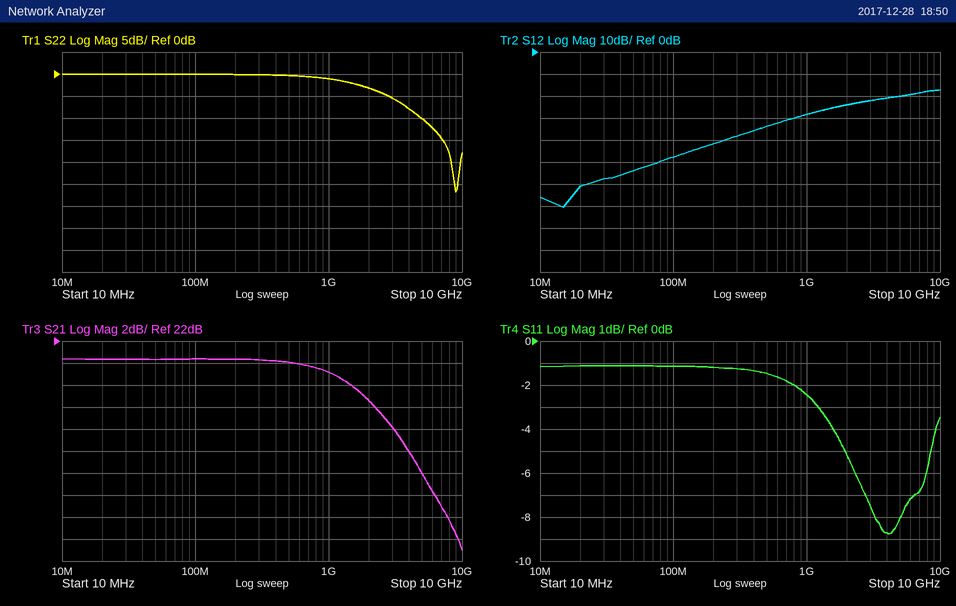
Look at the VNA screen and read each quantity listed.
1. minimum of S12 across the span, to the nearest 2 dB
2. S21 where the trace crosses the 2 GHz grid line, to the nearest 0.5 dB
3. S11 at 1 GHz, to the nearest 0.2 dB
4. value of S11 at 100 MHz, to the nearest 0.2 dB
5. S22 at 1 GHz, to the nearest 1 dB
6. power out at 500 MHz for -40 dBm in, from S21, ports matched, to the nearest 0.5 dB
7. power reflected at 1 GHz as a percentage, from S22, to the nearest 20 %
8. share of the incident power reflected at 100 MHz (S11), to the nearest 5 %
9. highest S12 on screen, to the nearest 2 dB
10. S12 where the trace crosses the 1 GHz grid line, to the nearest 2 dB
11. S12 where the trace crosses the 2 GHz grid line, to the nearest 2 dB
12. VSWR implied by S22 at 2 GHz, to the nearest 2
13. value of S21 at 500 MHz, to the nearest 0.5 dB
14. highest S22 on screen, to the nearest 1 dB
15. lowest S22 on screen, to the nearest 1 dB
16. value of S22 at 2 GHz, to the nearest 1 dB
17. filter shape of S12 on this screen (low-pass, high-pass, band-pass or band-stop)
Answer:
-70 dB
16.5 dB
-2.4 dB
-1.2 dB
-1 dB
-20.0 dBm
80 %
75 %
-18 dB
-28 dB
-24 dB
6
20.0 dB
0 dB
-27 dB
-3 dB
high-pass
